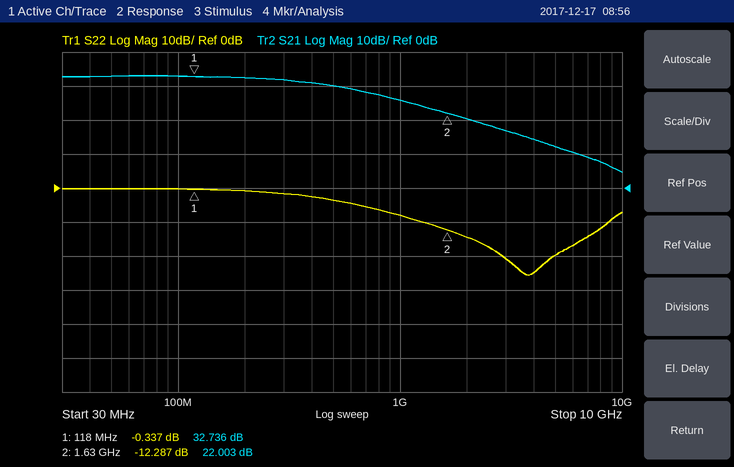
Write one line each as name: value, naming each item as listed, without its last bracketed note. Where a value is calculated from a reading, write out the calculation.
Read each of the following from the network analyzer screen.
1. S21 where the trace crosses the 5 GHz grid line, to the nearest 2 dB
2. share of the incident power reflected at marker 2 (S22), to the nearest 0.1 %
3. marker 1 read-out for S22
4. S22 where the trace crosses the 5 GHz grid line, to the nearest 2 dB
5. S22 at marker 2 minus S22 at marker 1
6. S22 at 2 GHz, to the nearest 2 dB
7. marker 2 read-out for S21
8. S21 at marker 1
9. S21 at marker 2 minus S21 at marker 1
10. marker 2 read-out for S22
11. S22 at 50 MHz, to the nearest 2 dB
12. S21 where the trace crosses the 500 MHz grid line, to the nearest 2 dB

S21 where the trace crosses the 5 GHz grid line, to the nearest 2 dB: 12 dB
share of the incident power reflected at marker 2 (S22), to the nearest 0.1 %: 10^(-12.287/10) ≈ 5.9 %
marker 1 read-out for S22: -0.337 dB
S22 where the trace crosses the 5 GHz grid line, to the nearest 2 dB: -20 dB
S22 at marker 2 minus S22 at marker 1: -12.287 − (-0.337) = -11.950 dB
S22 at 2 GHz, to the nearest 2 dB: -14 dB
marker 2 read-out for S21: 22.003 dB
S21 at marker 1: 32.736 dB
S21 at marker 2 minus S21 at marker 1: 22.003 − (32.736) = -10.733 dB
marker 2 read-out for S22: -12.287 dB
S22 at 50 MHz, to the nearest 2 dB: 0 dB
S21 where the trace crosses the 500 MHz grid line, to the nearest 2 dB: 30 dB
